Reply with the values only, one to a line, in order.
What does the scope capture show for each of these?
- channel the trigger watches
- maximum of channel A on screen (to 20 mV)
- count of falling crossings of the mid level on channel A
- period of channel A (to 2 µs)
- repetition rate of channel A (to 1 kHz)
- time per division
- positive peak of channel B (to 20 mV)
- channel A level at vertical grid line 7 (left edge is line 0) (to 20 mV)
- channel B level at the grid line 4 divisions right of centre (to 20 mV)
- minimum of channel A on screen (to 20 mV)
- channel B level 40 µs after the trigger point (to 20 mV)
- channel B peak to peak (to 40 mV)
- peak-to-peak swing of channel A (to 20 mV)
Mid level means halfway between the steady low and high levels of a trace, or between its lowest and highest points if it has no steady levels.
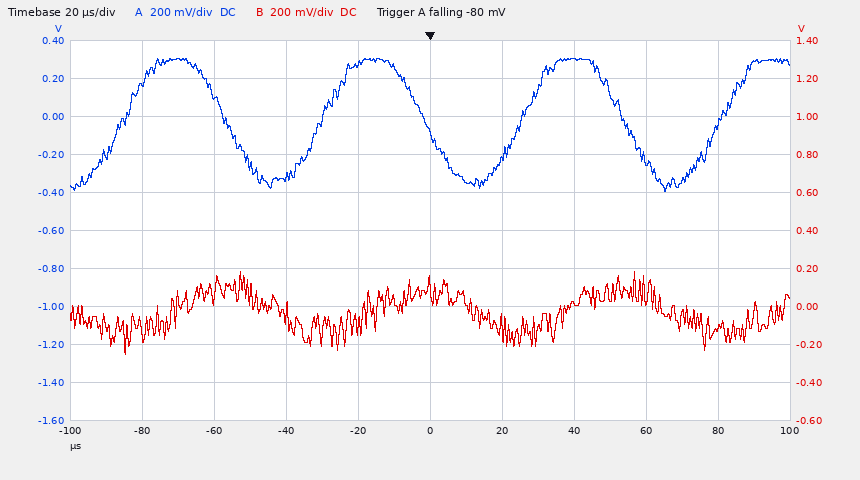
channel A
300 mV
3
56 µs
18 kHz
20 µs
180 mV
300 mV
-120 mV
-400 mV
20 mV
440 mV
700 mV
